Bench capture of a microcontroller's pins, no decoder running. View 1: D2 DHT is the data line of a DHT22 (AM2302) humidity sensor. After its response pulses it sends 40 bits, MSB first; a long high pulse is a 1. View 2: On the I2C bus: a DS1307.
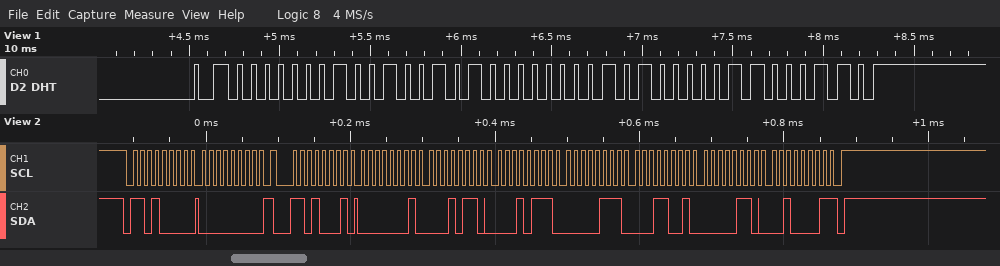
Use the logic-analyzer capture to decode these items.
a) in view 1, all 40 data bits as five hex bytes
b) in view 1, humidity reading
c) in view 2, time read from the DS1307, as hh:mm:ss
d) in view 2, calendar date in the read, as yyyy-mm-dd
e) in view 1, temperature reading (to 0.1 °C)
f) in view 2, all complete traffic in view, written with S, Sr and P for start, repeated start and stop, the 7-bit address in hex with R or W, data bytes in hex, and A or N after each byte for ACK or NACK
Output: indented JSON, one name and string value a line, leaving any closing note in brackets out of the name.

{
  "in view 1, all 40 data bits as five hex bytes": "01 25 00 A0 C6",
  "in view 1, humidity reading": "29.3 %",
  "in view 2, time read from the DS1307, as hh:mm:ss": "17:16:01",
  "in view 2, calendar date in the read, as yyyy-mm-dd": "2021-06-19",
  "in view 1, temperature reading": "16.0 °C",
  "in view 2, all complete traffic in view, written with S, Sr and P for start, repeated start and stop, the 7-bit address in hex with R or W, data bytes in hex, and A or N after each byte for ACK or NACK": "S 68W A 00 A Sr 68R A 01 A 16 A 17 A 07 A 19 A 06 A 21 N P"
}
